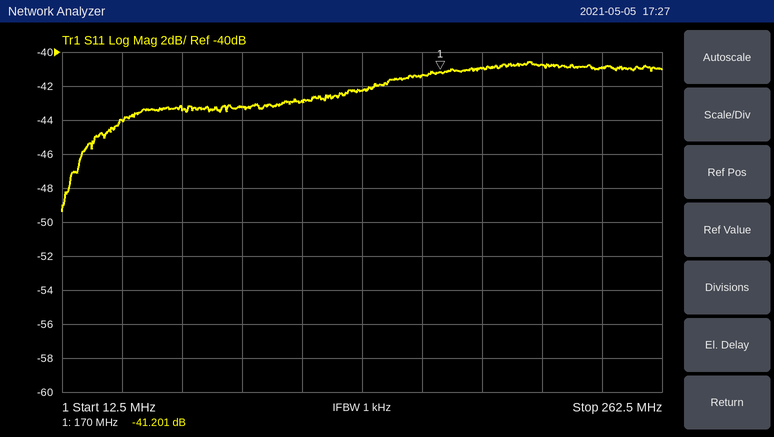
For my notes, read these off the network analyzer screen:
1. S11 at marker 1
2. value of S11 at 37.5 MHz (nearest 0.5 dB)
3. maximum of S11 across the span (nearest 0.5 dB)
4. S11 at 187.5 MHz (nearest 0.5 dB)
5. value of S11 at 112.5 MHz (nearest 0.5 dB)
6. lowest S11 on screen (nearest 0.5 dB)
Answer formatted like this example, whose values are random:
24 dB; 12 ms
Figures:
-41.201 dB; -44.0 dB; -40.5 dB; -41.0 dB; -43.0 dB; -49.5 dB
